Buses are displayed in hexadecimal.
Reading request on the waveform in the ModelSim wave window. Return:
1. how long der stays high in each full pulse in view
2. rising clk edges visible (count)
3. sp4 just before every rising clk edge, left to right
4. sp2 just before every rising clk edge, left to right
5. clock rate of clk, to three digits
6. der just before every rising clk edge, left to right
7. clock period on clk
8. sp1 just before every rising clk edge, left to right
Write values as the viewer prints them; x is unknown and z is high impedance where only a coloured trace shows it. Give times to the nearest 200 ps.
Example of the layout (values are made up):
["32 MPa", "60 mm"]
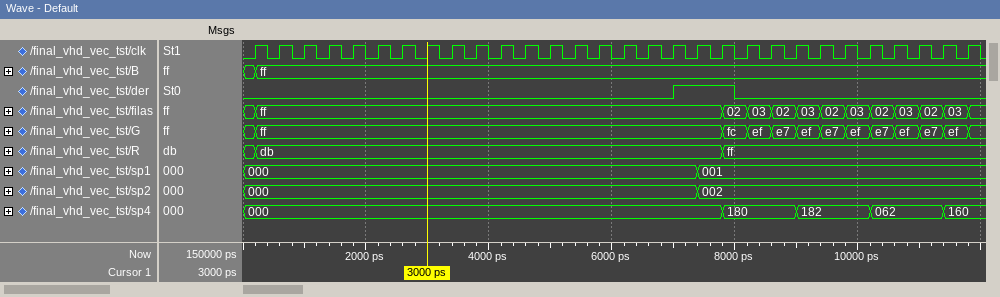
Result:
["1000 ps", "30", "000, 000, 000, 000, 000, 000, 000, 000, 000, 000, 000, 000, 000, 000, 000, 000, 000, 000, 000, 000, 180, 180, 180, 182, 182, 182, 062, 062, 062, 160", "000, 000, 000, 000, 000, 000, 000, 000, 000, 000, 000, 000, 000, 000, 000, 000, 000, 000, 000, 002, 002, 002, 002, 002, 002, 002, 002, 002, 002, 002", "2.50 GHz", "0 0 0 0 0 0 0 0 0 0 0 0 0 0 0 0 0 0 1 1 0 0 0 0 0 0 0 0 0 0", "400 ps", "000, 000, 000, 000, 000, 000, 000, 000, 000, 000, 000, 000, 000, 000, 000, 000, 000, 000, 000, 001, 001, 001, 001, 001, 001, 001, 001, 001, 001, 001"]
